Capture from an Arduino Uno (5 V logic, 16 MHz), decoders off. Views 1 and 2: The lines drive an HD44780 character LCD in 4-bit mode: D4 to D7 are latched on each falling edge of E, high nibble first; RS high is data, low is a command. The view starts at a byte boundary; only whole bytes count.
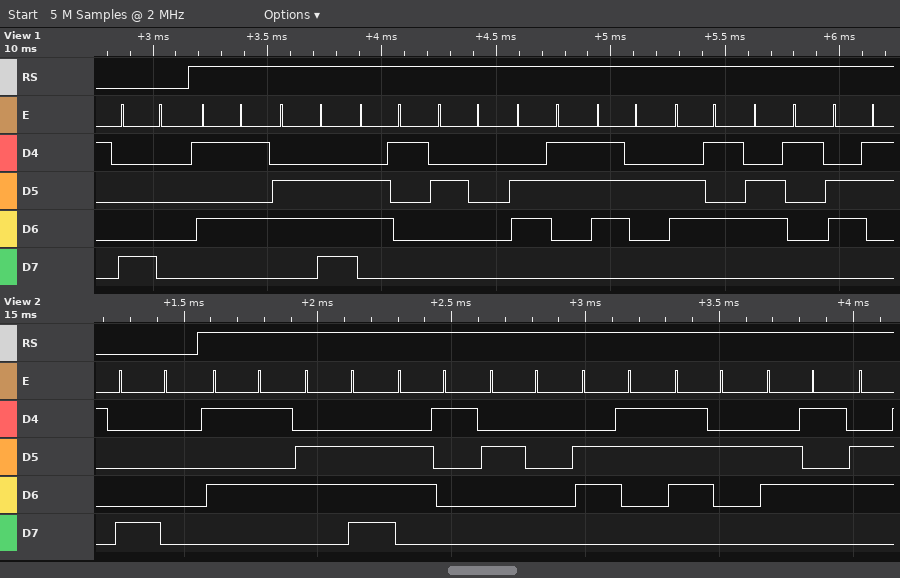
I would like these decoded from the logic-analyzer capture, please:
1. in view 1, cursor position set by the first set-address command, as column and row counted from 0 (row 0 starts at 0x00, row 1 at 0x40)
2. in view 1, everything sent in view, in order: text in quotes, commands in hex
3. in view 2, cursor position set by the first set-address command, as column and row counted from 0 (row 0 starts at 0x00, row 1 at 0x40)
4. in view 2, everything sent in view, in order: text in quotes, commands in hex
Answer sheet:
column 0, row 0
0x80 "Una creac"
column 0, row 0
0x80 "Una cre"
